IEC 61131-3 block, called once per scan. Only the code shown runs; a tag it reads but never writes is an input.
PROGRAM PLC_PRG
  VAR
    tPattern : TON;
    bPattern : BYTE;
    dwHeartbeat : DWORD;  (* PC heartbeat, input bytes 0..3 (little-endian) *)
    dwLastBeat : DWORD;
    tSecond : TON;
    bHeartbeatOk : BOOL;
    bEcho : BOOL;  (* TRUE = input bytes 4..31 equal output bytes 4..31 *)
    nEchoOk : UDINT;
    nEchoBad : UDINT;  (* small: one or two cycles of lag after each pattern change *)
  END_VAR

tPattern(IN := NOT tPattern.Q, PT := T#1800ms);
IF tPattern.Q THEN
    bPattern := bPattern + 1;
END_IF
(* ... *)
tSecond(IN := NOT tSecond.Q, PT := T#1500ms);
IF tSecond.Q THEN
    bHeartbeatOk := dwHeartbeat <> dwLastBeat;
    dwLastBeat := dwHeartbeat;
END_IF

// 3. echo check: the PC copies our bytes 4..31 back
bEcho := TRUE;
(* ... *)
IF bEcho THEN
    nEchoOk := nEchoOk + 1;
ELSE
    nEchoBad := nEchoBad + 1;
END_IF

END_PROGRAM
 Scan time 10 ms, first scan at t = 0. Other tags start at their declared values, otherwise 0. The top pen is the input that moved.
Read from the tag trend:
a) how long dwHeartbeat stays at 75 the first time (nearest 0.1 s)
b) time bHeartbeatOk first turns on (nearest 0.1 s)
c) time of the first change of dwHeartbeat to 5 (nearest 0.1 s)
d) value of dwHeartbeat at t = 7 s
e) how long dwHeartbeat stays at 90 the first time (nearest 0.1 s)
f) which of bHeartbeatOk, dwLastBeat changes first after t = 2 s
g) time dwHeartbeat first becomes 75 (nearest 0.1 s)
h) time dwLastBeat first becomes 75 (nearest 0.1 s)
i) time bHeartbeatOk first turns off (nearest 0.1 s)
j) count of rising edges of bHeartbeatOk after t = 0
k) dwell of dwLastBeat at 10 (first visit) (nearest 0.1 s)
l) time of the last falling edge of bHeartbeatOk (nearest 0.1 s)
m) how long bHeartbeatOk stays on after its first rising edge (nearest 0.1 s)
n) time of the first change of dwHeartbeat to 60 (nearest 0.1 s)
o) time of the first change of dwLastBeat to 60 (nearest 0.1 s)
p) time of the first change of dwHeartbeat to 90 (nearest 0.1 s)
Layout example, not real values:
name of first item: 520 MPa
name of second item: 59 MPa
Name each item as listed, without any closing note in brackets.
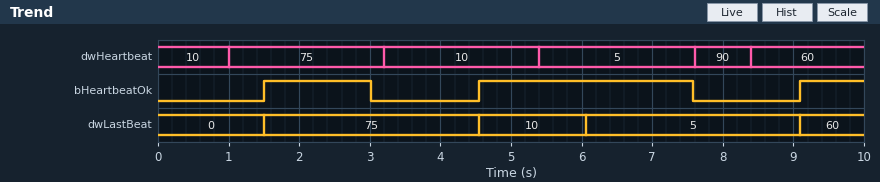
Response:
how long dwHeartbeat stays at 75 the first time: 2.2 s
time bHeartbeatOk first turns on: 1.5 s
time of the first change of dwHeartbeat to 5: 5.4 s
value of dwHeartbeat at t = 7 s: 5
how long dwHeartbeat stays at 90 the first time: 0.8 s
which of bHeartbeatOk, dwLastBeat changes first after t = 2 s: bHeartbeatOk
time dwHeartbeat first becomes 75: 1.0 s
time dwLastBeat first becomes 75: 1.5 s
time bHeartbeatOk first turns off: 3.0 s
count of rising edges of bHeartbeatOk after t = 0: 3
dwell of dwLastBeat at 10 (first visit): 1.5 s
time of the last falling edge of bHeartbeatOk: 7.6 s
how long bHeartbeatOk stays on after its first rising edge: 1.5 s
time of the first change of dwHeartbeat to 60: 8.4 s
time of the first change of dwLastBeat to 60: 9.1 s
time of the first change of dwHeartbeat to 90: 7.6 s
